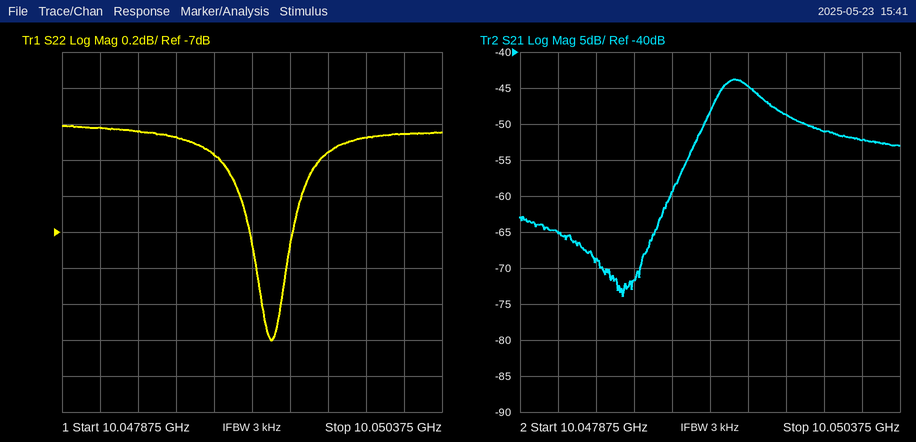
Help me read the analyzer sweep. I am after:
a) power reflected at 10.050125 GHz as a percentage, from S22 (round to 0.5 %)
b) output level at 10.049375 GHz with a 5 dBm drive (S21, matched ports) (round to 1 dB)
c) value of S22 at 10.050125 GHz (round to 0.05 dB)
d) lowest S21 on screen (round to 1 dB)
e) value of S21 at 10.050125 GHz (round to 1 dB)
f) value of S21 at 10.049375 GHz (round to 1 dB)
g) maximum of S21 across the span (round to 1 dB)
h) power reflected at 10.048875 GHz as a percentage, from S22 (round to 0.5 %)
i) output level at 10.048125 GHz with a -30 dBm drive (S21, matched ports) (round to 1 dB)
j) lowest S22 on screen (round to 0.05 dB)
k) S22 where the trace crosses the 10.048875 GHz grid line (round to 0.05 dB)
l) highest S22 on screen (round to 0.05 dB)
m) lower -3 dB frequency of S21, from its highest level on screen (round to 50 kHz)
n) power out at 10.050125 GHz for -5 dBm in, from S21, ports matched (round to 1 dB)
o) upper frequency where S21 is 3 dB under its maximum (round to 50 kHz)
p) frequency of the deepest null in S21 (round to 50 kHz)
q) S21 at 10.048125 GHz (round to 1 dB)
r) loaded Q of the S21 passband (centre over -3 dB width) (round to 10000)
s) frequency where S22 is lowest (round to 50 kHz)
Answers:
22.5 %
-40 dBm
-6.45 dB
-74 dB
-52 dB
-45 dB
-44 dB
22.0 %
-95 dBm
-7.60 dB
-6.55 dB
-6.40 dB
10.04915 GHz
-57 dBm
10.04950 GHz
10.04855 GHz
-65 dB
30000
10.04925 GHz
